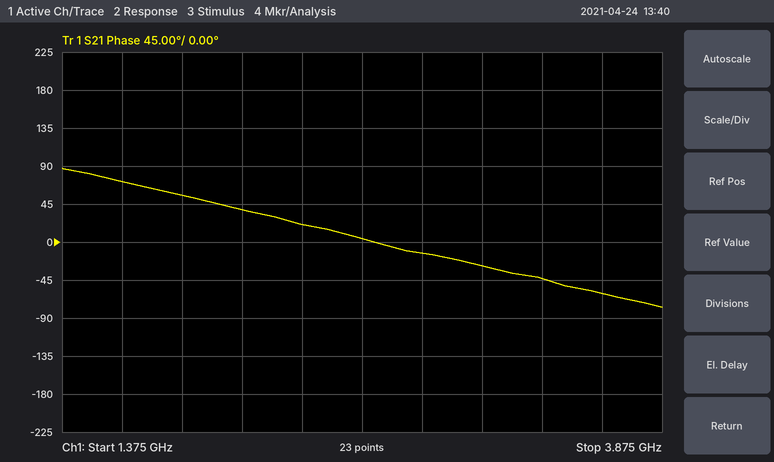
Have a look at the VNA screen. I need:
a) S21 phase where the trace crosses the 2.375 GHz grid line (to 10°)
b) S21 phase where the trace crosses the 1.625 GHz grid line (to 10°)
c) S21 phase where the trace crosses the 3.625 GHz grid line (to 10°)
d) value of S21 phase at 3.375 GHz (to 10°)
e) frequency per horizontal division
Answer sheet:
20°
70°
-60°
-40°
250 MHz
